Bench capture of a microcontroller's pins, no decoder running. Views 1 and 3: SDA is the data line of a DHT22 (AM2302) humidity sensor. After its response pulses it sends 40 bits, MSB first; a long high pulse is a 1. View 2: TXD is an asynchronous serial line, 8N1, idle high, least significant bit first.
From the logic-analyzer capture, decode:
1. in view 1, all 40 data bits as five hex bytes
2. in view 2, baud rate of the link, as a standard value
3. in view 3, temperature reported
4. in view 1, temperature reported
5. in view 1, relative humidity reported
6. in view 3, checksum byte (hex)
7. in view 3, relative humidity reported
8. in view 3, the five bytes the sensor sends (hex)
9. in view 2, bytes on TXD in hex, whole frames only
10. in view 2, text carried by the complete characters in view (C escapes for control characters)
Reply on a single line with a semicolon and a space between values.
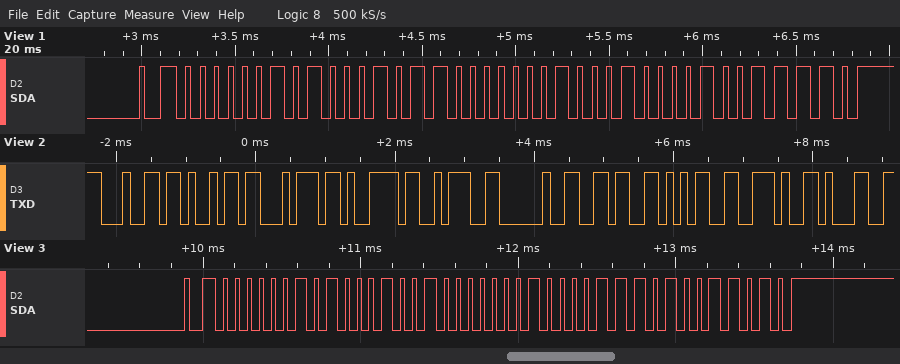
02 8B 01 10 9E; 9600 baud; 27.0 °C; 27.2 °C; 65.1 %; 0x9A; 64.9 %; 02 89 01 0E 9A; 64 69 74 79 3A 20 36 35 2E 31; "dity: 65.1"
